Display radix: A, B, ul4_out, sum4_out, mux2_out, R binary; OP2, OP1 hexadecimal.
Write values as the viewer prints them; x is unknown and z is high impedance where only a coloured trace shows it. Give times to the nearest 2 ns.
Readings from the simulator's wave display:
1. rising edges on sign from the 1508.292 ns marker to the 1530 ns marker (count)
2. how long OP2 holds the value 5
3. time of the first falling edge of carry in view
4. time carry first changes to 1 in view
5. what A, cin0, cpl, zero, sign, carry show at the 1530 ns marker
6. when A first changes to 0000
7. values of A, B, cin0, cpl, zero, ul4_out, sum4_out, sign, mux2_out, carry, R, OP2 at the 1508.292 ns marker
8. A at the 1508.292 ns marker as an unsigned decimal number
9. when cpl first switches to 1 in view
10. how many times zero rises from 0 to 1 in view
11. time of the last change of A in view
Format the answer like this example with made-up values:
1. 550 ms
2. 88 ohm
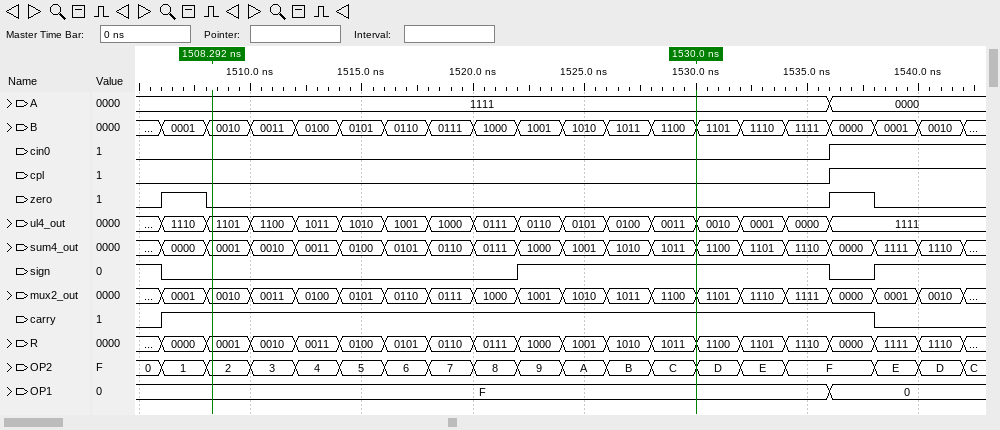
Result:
1. 1
2. 2 ns
3. 1538 ns
4. 1506 ns
5. A=1111, cin0=0, cpl=0, zero=0, sign=1, carry=1
6. 1536 ns
7. A=1111, B=0010, cin0=0, cpl=0, zero=0, ul4_out=1101, sum4_out=0001, sign=0, mux2_out=0010, carry=1, R=0001, OP2=2
8. 15
9. 1536 ns
10. 2
11. 1536 ns
